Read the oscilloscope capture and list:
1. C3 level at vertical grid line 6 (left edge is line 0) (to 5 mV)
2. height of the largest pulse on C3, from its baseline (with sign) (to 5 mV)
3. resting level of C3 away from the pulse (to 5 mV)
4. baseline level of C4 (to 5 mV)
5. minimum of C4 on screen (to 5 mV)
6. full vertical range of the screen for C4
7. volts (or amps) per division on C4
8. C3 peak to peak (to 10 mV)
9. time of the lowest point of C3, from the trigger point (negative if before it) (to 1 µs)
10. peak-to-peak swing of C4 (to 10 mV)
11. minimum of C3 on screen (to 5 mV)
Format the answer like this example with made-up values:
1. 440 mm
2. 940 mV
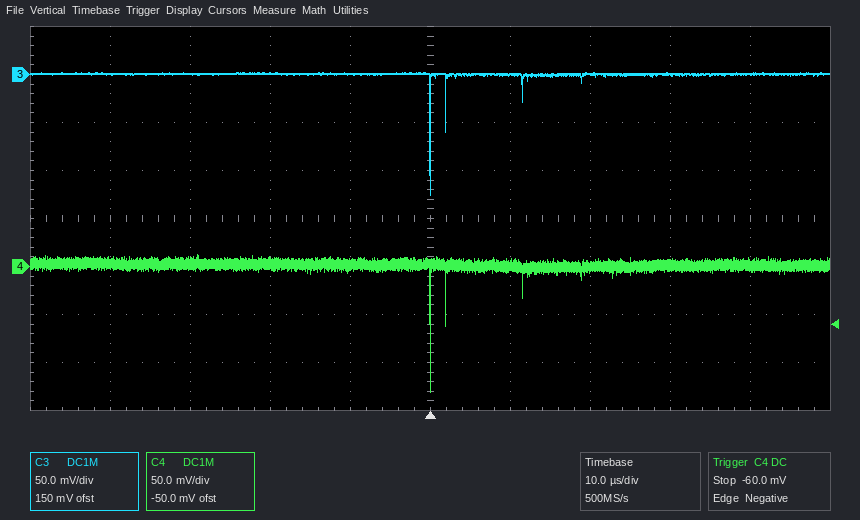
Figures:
1. 0 mV
2. -125 mV
3. 0 mV
4. 0 mV
5. -130 mV
6. 400 mV
7. 50 mV
8. 130 mV
9. 0 µs
10. 140 mV
11. -125 mV
